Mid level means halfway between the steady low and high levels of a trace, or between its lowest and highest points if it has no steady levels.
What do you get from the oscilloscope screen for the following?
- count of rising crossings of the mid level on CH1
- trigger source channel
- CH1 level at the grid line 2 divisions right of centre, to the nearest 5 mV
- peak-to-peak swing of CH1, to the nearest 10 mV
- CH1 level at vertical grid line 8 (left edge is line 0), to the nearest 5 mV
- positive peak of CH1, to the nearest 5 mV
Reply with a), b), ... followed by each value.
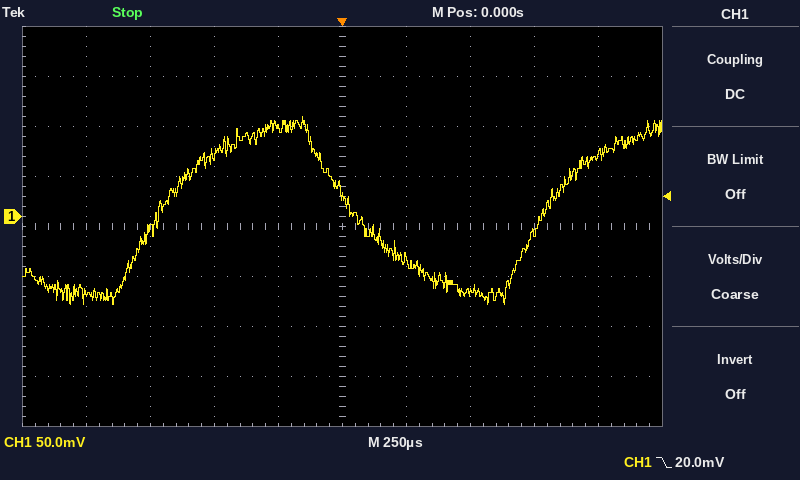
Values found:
a) 2
b) CH1
c) -75 mV
d) 190 mV
e) -15 mV
f) 100 mV
